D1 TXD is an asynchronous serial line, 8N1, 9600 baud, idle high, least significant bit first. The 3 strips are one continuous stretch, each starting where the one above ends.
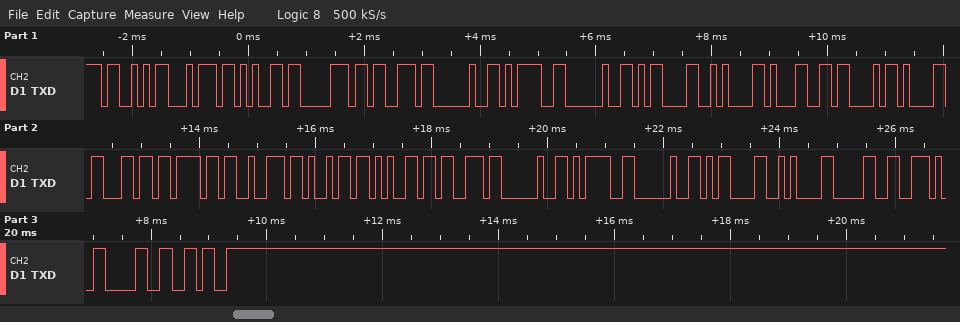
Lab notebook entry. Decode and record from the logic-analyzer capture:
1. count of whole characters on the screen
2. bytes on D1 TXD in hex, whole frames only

28
53 74 65 70 73 20 3D 20 0D 0A 31 43 61 6C 6F 72 69 65 73 20 3D 20 0D 0A 30 2E 30 36
